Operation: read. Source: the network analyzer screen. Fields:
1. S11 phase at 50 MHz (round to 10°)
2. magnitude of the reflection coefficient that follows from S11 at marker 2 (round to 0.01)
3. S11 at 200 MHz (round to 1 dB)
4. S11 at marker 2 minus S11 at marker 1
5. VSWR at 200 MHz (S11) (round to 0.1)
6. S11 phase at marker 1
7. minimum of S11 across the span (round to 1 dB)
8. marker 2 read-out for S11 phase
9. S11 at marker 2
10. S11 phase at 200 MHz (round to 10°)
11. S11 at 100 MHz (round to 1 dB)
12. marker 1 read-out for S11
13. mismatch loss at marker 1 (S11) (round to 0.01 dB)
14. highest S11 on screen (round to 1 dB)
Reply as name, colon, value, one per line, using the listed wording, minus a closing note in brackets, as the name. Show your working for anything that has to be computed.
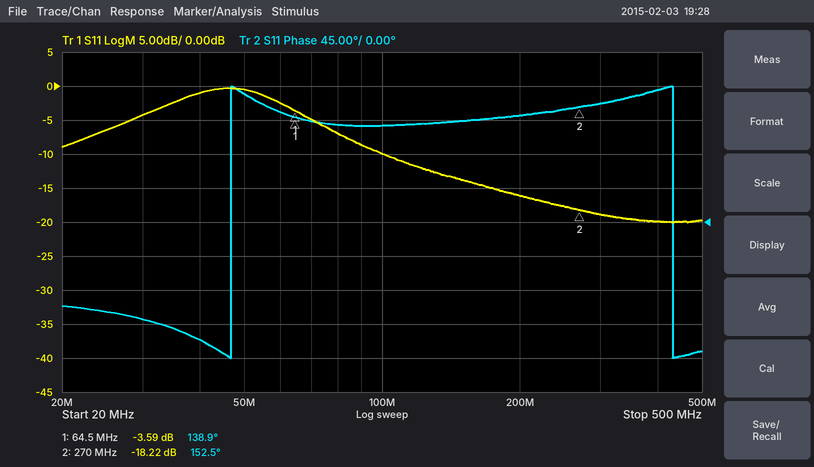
S11 phase at 50 MHz: 170°
magnitude of the reflection coefficient that follows from S11 at marker 2: 10^(-18.22/20) ≈ 0.12
S11 at 200 MHz: -16 dB
S11 at marker 2 minus S11 at marker 1: -18.22 − (-3.59) = -14.63 dB
VSWR at 200 MHz (S11): |Γ| = 10^(-16/20) = 0.1585; VSWR = (1 + 0.1585)/(1 − 0.1585) ≈ 1.4
S11 phase at marker 1: 138.9°
minimum of S11 across the span: -20 dB
marker 2 read-out for S11 phase: 152.5°
S11 at marker 2: -18.22 dB
S11 phase at 200 MHz: 140°
S11 at 100 MHz: -10 dB
marker 1 read-out for S11: -3.59 dB
mismatch loss at marker 1 (S11): −10 log10(1 − 10^(-3.59/10)) ≈ 2.50 dB
highest S11 on screen: 0 dB
